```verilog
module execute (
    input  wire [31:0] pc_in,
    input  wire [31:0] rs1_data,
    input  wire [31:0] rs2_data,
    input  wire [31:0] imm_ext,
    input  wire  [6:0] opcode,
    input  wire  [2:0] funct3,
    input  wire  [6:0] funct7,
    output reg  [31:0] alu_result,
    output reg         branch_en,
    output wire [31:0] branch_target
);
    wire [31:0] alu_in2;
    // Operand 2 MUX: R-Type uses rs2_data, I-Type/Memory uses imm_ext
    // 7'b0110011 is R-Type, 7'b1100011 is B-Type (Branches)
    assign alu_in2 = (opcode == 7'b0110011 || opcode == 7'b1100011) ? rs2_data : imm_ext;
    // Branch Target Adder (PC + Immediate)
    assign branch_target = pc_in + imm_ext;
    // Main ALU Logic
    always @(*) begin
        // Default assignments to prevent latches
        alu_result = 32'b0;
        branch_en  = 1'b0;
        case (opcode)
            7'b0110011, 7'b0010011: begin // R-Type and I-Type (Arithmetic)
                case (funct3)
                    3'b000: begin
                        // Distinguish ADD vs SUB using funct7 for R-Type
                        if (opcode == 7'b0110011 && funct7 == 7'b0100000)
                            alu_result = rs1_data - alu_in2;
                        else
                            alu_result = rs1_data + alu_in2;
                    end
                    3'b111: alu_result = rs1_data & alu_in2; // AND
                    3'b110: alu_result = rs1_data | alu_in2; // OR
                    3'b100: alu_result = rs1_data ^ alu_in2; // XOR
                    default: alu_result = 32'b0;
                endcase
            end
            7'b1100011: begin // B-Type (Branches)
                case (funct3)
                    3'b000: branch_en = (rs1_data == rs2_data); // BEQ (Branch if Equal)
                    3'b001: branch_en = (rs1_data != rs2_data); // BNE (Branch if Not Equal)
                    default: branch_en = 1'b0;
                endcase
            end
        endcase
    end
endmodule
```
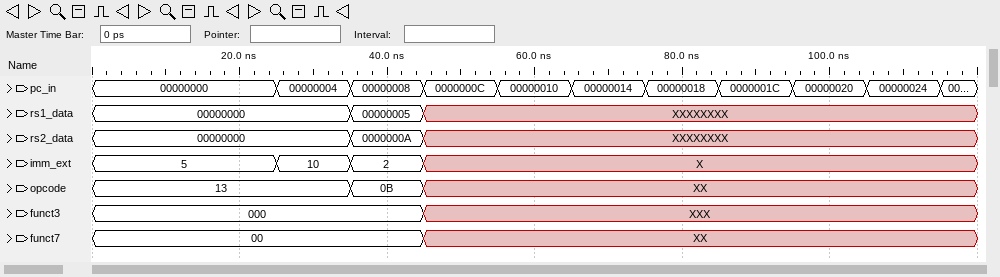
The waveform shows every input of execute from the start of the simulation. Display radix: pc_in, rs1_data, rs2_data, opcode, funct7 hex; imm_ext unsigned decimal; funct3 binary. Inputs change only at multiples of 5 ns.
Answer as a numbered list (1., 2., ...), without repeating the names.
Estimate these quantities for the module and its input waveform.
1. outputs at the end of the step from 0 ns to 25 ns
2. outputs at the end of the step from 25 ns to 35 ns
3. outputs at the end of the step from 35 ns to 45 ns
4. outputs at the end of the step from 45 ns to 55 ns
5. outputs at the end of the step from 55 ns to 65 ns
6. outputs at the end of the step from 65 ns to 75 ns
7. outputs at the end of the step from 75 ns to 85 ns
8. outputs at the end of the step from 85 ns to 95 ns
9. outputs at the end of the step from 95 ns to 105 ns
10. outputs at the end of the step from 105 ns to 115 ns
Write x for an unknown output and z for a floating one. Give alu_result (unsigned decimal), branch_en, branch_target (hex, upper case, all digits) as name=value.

1. alu_result=5, branch_en=0, branch_target=00000005
2. alu_result=10, branch_en=0, branch_target=0000000E
3. alu_result=0, branch_en=0, branch_target=0000000A
4. alu_result=0, branch_en=0, branch_target=x
5. alu_result=0, branch_en=0, branch_target=x
6. alu_result=0, branch_en=0, branch_target=x
7. alu_result=0, branch_en=0, branch_target=x
8. alu_result=0, branch_en=0, branch_target=x
9. alu_result=0, branch_en=0, branch_target=x
10. alu_result=0, branch_en=0, branch_target=x
